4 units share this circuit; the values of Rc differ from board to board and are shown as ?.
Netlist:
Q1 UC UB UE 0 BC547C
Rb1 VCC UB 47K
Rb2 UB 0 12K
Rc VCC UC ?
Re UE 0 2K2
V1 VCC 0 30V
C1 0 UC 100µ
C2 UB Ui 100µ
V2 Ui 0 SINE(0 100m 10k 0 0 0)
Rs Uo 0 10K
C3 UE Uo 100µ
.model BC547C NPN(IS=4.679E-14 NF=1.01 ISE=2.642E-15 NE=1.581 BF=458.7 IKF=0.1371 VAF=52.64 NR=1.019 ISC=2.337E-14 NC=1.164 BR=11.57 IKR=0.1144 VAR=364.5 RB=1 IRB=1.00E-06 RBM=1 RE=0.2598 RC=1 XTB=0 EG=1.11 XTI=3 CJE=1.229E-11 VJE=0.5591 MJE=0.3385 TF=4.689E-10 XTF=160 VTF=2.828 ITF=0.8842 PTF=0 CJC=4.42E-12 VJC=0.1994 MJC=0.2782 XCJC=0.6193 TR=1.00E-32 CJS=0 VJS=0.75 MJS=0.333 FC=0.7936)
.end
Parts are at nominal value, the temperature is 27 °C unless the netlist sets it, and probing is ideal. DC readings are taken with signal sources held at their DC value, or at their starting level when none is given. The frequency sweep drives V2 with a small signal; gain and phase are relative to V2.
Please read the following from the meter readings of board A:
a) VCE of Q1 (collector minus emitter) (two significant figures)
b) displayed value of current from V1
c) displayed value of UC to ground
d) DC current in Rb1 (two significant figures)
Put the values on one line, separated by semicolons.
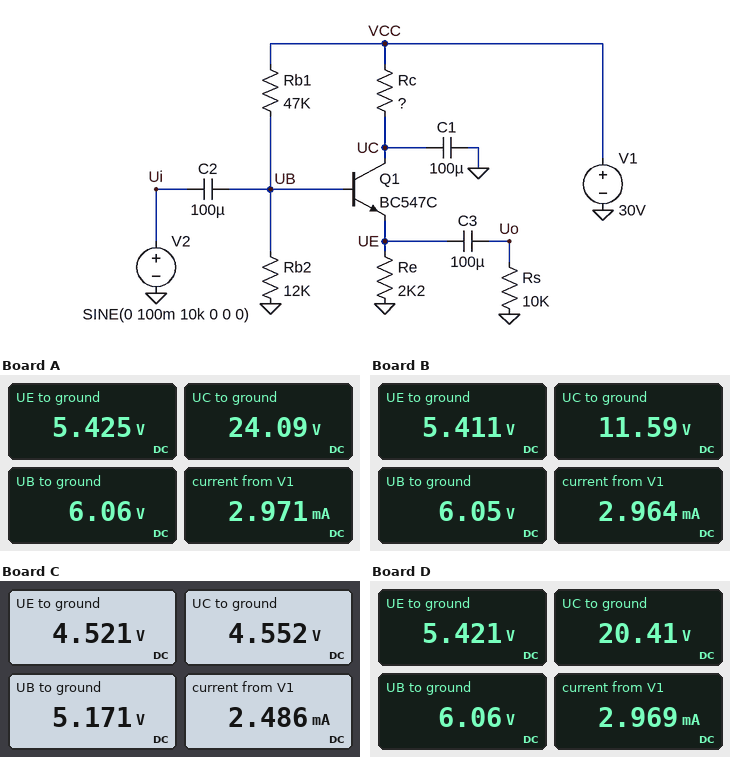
19 V; 2.971 mA; 24.09 V; 510 µA
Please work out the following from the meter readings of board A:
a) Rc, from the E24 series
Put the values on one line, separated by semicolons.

2.4 kΩ
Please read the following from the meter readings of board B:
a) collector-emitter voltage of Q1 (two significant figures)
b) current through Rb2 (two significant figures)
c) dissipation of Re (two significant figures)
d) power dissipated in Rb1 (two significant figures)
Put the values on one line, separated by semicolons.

6.2 V; 500 µA; 13 mW; 12 mW
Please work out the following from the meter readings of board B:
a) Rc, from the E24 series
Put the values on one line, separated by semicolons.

7.5 kΩ
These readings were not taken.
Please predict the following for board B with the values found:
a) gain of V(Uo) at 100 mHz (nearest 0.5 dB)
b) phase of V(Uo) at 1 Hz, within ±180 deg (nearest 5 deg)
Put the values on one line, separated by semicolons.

-11.5 dB; 20 deg
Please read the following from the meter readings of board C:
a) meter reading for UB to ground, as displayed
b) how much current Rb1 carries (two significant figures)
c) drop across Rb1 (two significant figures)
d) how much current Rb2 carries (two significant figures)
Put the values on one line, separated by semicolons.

5.171 V; 530 µA; 25 V; 430 µA
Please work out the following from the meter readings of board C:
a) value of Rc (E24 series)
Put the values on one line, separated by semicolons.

13 kΩ
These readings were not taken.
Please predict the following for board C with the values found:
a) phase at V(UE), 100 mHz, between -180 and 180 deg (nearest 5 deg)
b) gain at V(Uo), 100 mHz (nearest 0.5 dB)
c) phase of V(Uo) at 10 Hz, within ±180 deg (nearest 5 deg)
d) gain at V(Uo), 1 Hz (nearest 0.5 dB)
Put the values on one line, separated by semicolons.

75 deg; -26.0 dB; 15 deg; -7.5 dB
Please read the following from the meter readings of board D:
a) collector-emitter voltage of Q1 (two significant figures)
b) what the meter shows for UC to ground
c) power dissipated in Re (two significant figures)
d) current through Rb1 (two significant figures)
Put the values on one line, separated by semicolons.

15 V; 20.41 V; 13 mW; 510 µA
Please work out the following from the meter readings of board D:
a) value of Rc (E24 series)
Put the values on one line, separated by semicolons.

3.9 kΩ
